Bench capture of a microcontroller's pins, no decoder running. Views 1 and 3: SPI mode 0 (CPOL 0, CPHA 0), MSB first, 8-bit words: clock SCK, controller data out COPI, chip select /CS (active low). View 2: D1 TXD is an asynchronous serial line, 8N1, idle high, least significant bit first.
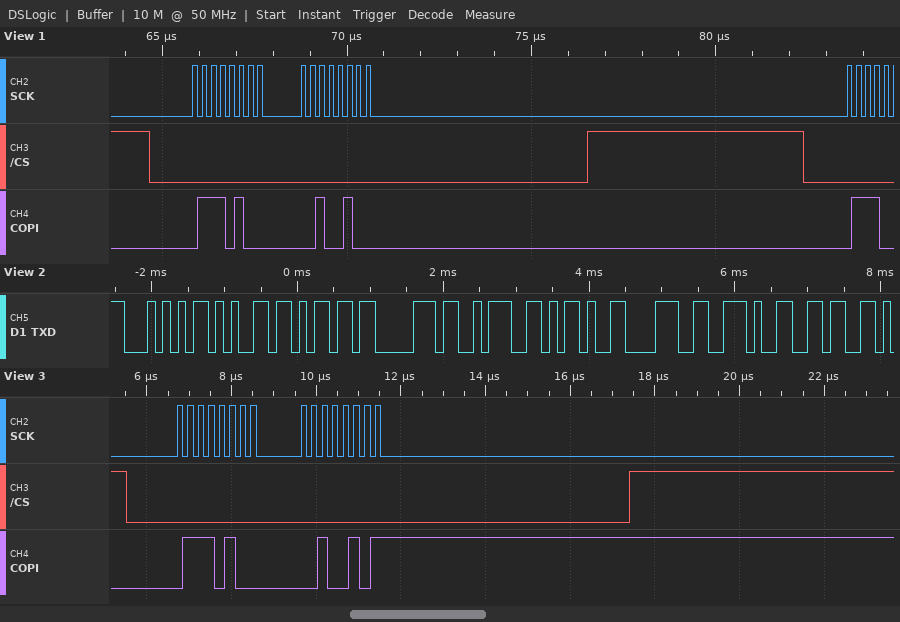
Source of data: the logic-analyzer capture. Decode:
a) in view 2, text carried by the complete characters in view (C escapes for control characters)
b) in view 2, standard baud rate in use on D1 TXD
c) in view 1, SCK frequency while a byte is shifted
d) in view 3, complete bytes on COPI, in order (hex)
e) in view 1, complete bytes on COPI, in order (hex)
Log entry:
"Temp:-8.6"
9600 baud
4 MHz
74 25
74 24
